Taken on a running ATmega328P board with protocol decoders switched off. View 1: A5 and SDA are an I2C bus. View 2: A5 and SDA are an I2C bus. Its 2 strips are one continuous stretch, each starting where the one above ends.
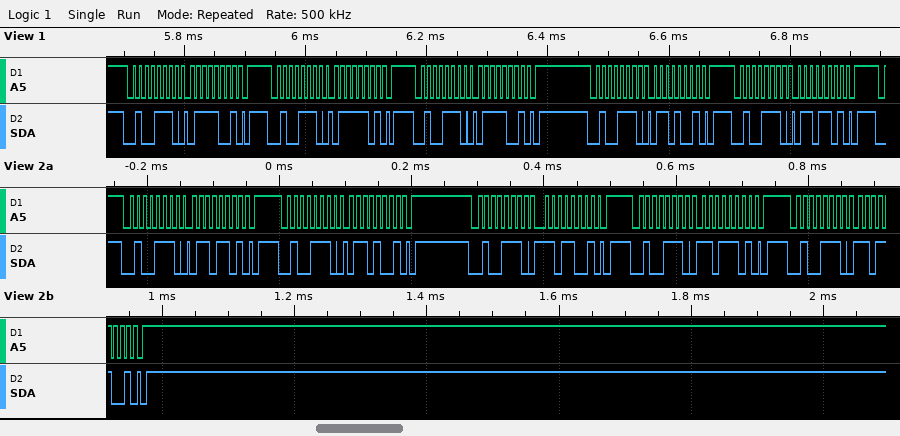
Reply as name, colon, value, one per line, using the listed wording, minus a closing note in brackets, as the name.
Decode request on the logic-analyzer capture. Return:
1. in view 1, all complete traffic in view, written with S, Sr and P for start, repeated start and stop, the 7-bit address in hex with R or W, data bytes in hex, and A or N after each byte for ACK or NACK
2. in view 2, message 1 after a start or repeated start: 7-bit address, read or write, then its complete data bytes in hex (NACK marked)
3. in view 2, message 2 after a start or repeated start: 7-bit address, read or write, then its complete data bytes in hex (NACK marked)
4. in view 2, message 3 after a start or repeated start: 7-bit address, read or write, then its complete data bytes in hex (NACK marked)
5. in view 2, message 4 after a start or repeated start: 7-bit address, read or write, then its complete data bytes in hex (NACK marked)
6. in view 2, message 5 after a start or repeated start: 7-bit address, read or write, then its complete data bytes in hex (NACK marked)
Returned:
in view 1, all complete traffic in view, written with S, Sr and P for start, repeated start and stop, the 7-bit address in hex with R or W, data bytes in hex, and A or N after each byte for ACK or NACK: S 27W A 79 A P S 27W A 7D A P S 27W A 79 A P S 27W A 69 A P S 27W A 6D A P
in view 2, message 1 after a start or repeated start: 7-bit address, read or write, then its complete data bytes in hex: 0x27 write: 6D
in view 2, message 2 after a start or repeated start: 7-bit address, read or write, then its complete data bytes in hex: 0x27 write: 69
in view 2, message 3 after a start or repeated start: 7-bit address, read or write, then its complete data bytes in hex: 0x27 write: D9
in view 2, message 4 after a start or repeated start: 7-bit address, read or write, then its complete data bytes in hex: 0x27 write: DD
in view 2, message 5 after a start or repeated start: 7-bit address, read or write, then its complete data bytes in hex: 0x27 write: D9
